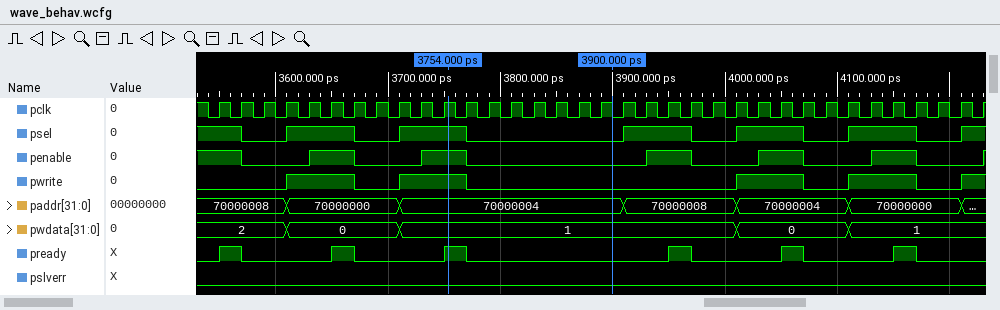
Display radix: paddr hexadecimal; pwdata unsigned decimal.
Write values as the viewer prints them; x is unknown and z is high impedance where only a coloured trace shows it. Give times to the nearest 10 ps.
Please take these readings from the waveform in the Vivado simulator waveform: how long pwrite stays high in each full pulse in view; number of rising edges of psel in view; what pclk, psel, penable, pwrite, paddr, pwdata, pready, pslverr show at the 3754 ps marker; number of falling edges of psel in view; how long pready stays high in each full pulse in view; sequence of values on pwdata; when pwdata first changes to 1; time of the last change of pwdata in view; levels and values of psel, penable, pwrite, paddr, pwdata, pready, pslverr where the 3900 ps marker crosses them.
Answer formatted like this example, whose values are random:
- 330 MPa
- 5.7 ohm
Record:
- 60 ps, 60 ps, 60 ps, 60 ps
- 6
- pclk=1, psel=1, penable=1, pwrite=1, paddr=70000004, pwdata=1, pready=1, pslverr=0
- 6
- 20 ps, 20 ps, 20 ps, 20 ps, 20 ps, 20 ps
- 2, 0, 1, 0, 1
- 3710 ps
- 4110 ps
- psel=0, penable=0, pwrite=0, paddr=70000004, pwdata=1, pready=0, pslverr=0
